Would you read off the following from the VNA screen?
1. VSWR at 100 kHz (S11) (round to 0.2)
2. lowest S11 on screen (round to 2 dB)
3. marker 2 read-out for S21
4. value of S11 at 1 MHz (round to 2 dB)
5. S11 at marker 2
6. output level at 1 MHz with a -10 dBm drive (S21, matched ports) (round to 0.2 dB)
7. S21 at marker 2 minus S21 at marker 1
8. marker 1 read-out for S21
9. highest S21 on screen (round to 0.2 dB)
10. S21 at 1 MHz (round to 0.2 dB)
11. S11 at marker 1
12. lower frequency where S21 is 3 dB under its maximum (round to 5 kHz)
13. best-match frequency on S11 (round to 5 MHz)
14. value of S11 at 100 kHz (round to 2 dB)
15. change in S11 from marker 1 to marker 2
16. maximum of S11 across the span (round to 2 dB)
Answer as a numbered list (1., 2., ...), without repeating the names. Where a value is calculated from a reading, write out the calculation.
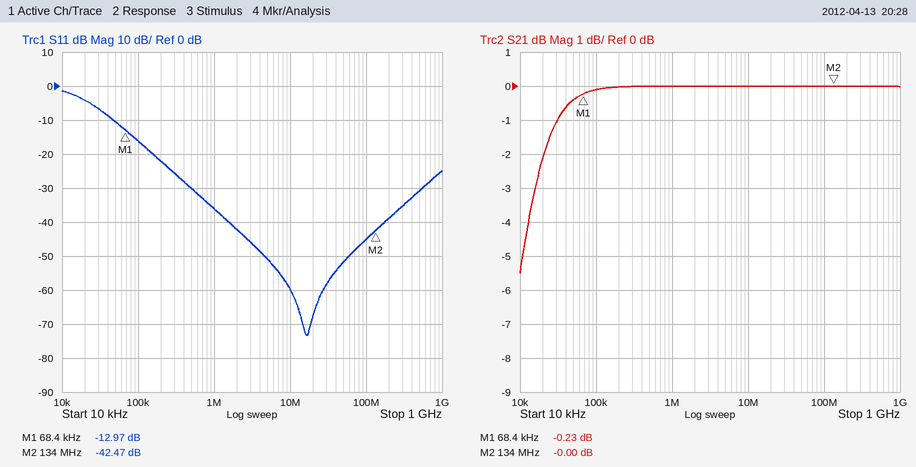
1. |Γ| = 10^(-16/20) = 0.1585; VSWR = (1 + 0.1585)/(1 − 0.1585) ≈ 1.4
2. -74 dB
3. -0.00 dB
4. -36 dB
5. -42.47 dB
6. -10 dBm + (0.0 dB) = -10.0 dBm
7. -0 − (-0.23) = 0.23 dB
8. -0.23 dB
9. 0.0 dB
10. 0.0 dB
11. -12.97 dB
12. 15 kHz
13. 15 MHz
14. -16 dB
15. -42.47 − (-12.97) = -29.50 dB
16. -2 dB
